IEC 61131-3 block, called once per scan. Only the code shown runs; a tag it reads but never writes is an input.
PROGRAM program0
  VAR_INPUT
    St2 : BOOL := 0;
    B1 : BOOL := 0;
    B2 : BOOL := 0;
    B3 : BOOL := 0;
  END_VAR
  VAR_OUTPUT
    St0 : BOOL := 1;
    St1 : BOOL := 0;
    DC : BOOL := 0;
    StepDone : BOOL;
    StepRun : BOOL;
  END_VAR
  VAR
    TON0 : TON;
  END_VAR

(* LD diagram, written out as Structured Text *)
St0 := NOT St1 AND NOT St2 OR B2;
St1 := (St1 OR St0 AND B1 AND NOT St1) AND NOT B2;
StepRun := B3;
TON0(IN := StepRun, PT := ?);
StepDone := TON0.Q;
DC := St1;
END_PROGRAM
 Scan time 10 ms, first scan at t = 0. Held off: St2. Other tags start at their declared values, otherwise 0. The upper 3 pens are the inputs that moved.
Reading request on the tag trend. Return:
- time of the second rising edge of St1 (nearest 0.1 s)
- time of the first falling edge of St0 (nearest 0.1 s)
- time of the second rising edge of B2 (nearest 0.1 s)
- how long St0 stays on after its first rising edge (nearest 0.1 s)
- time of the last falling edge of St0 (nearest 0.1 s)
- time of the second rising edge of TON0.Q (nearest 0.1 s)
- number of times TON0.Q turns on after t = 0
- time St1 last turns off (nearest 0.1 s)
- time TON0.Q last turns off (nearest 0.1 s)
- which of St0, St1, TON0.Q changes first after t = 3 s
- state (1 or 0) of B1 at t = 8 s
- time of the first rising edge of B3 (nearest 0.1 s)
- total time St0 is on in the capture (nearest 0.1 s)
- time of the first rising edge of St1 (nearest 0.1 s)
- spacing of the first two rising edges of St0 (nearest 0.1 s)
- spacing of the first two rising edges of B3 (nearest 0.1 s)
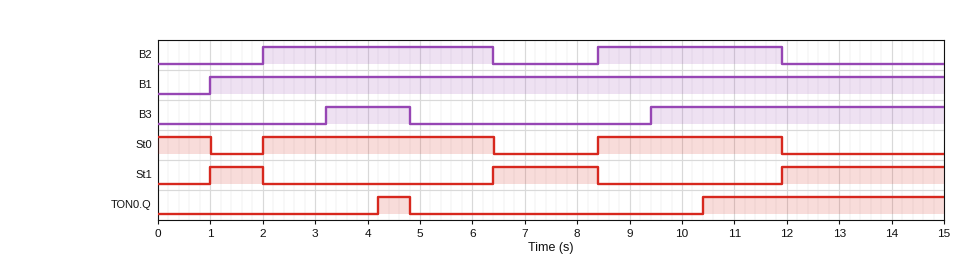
6.4 s
1.0 s
8.4 s
4.4 s
11.9 s
10.4 s
2
8.4 s
4.8 s
TON0.Q
1
3.2 s
8.9 s
1.0 s
6.4 s
6.2 s
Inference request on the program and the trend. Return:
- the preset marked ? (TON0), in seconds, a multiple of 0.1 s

1.0 s
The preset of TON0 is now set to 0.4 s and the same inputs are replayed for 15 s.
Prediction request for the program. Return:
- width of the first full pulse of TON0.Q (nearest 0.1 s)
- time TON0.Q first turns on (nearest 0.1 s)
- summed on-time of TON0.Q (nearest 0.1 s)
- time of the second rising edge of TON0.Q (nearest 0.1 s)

1.2 s
3.6 s
6.4 s
9.8 s
